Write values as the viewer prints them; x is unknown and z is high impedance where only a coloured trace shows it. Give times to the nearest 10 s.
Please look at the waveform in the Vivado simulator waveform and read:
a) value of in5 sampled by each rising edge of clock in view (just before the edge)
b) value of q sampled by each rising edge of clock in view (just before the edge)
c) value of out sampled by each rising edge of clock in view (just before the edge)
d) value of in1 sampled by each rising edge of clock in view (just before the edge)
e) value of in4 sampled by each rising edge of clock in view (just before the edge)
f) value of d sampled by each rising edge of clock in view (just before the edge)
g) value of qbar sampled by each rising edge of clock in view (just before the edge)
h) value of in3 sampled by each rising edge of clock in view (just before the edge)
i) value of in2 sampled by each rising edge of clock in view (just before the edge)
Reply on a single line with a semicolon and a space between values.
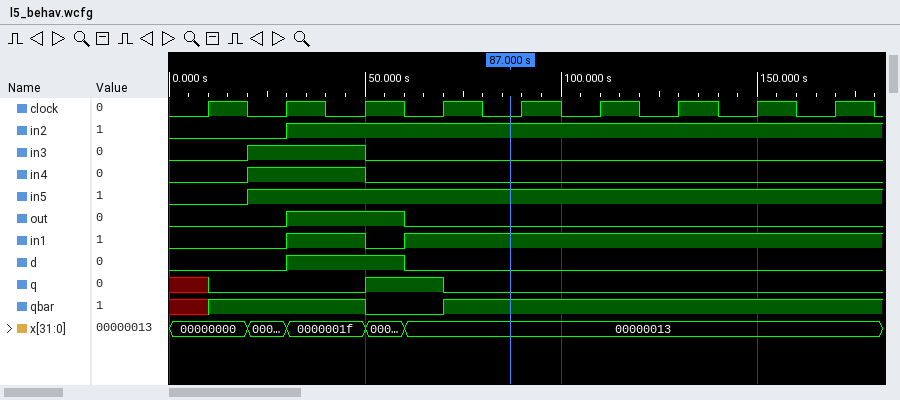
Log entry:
0 1 1 1 1 1 1 1 1; x 0 0 1 0 0 0 0 0; 0 0 1 0 0 0 0 0 0; 0 0 1 1 1 1 1 1 1; 0 1 1 0 0 0 0 0 0; 0 0 1 0 0 0 0 0 0; x 1 1 0 1 1 1 1 1; 0 1 1 0 0 0 0 0 0; 0 0 1 1 1 1 1 1 1
